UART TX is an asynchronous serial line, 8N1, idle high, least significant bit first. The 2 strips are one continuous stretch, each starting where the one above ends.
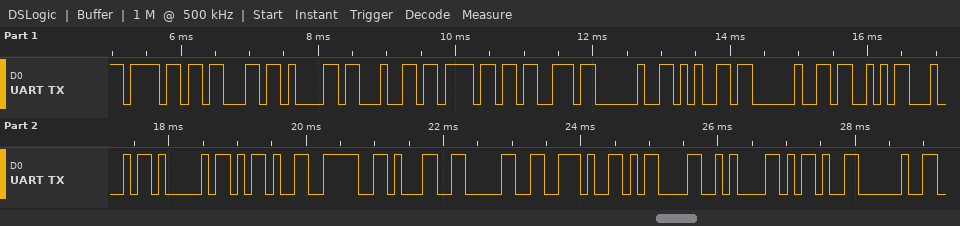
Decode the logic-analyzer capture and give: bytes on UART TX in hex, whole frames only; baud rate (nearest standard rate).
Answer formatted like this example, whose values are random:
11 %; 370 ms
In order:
6F 63 61 64 6F 73 20 65 20 53 44 41 2D 3E 31 30 2E 0D 0A 2D 20; 9600 baud
